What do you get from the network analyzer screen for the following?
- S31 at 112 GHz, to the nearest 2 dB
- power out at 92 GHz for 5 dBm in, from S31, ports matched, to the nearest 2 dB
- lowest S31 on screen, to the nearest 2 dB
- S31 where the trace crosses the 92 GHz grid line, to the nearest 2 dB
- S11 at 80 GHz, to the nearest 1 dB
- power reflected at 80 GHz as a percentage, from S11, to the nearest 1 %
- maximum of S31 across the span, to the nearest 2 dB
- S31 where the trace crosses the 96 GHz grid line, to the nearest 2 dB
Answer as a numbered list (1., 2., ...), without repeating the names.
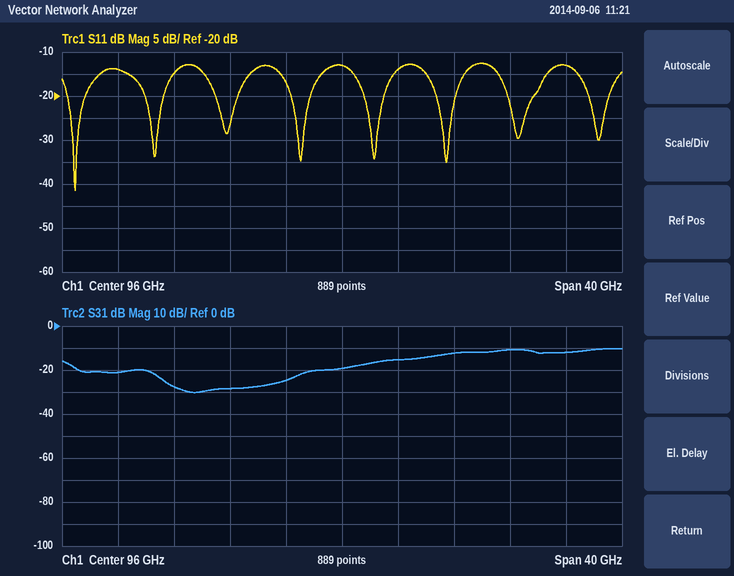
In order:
1. -12 dB
2. -20 dBm
3. -30 dB
4. -24 dB
5. -14 dB
6. 4 %
7. -10 dB
8. -20 dB
